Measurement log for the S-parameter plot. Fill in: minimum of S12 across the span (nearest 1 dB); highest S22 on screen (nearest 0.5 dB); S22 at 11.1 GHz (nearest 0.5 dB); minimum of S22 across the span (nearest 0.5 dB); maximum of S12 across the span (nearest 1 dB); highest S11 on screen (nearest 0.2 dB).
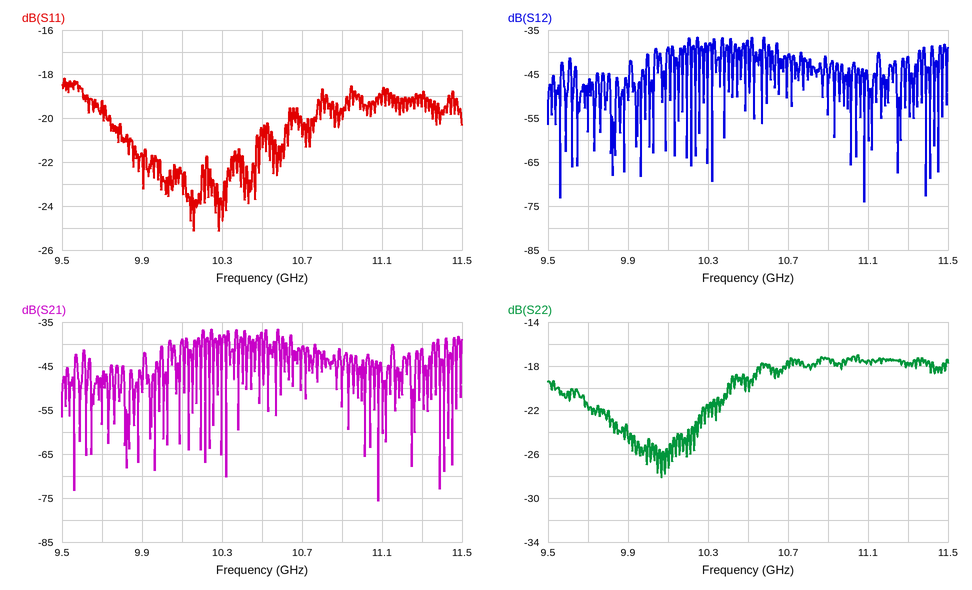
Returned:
-74 dB
-17.0 dB
-17.5 dB
-28.0 dB
-37 dB
-18.2 dB
